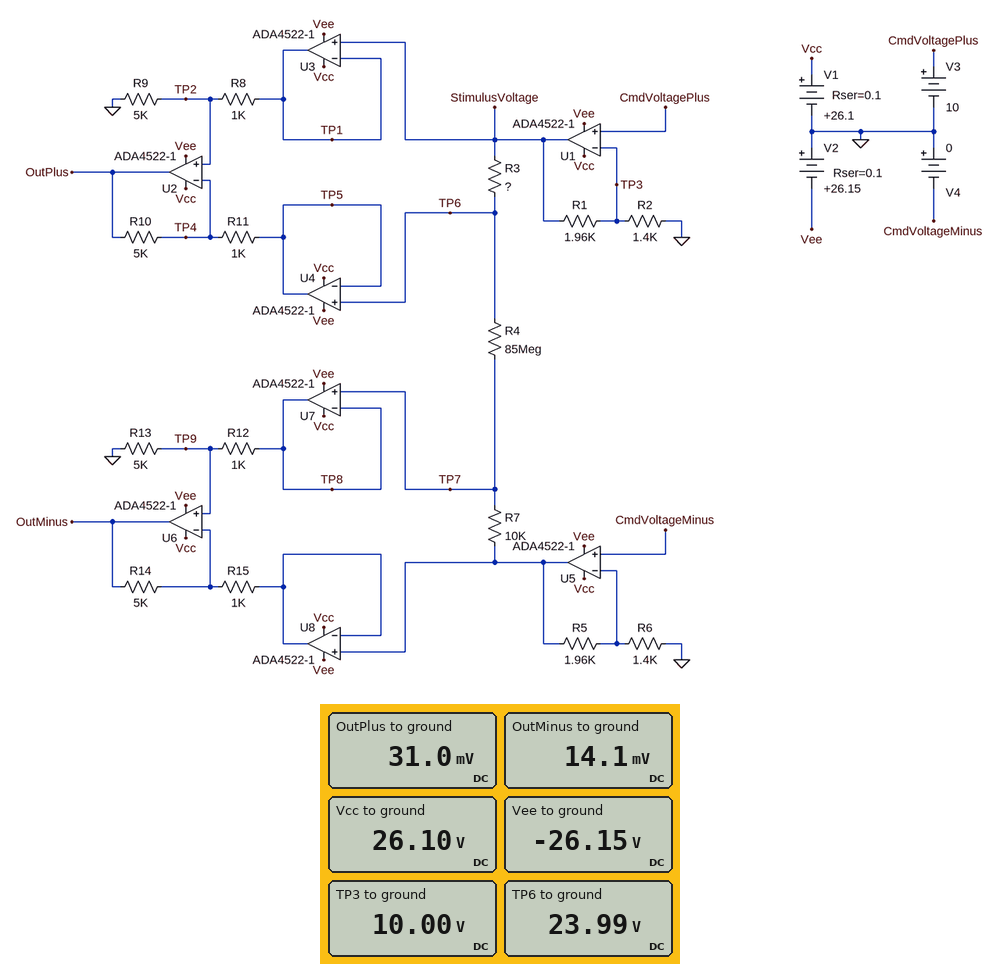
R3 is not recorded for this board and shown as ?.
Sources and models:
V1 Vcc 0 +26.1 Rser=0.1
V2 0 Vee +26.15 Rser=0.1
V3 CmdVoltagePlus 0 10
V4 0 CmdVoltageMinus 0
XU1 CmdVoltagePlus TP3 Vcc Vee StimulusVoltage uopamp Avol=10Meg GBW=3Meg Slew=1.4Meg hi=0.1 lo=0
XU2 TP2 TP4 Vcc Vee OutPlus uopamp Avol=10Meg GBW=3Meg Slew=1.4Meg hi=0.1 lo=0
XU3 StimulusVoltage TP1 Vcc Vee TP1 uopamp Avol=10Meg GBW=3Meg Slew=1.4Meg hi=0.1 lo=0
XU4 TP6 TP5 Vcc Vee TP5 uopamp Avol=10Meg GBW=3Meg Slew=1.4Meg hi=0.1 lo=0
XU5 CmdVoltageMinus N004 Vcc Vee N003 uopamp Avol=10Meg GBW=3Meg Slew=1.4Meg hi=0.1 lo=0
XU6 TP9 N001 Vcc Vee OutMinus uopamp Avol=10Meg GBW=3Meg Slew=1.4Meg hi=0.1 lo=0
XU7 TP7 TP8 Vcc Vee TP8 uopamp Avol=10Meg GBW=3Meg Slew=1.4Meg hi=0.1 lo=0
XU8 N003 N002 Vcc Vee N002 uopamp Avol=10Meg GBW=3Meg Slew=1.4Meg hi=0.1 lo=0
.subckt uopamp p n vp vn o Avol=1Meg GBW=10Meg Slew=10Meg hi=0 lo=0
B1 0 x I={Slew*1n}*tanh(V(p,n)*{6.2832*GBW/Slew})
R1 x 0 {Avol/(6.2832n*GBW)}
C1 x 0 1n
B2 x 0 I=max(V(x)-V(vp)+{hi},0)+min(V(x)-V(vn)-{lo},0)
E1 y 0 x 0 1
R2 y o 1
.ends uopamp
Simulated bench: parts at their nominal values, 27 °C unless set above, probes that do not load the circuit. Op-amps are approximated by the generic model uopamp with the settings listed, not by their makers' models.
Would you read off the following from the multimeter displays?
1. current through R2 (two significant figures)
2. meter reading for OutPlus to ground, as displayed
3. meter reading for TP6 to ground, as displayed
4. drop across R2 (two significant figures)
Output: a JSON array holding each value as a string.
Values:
["7.1 mA", "31.0 mV", "23.99 V", "10 V"]
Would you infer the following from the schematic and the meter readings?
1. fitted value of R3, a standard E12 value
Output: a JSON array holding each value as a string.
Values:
["22 kΩ"]
